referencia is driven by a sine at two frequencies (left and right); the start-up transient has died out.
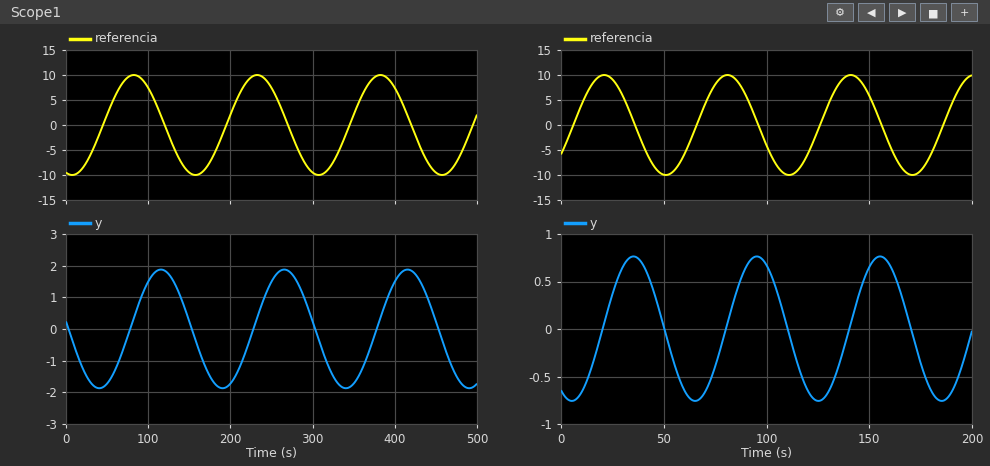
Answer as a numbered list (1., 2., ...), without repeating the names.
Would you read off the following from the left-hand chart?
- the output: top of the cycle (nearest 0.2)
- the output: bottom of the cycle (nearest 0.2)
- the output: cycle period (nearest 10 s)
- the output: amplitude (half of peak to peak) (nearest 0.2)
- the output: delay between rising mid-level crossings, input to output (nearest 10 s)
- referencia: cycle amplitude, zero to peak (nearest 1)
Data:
1. 1.8
2. -1.8
3. 150 s
4. 1.8
5. 30 s
6. 10
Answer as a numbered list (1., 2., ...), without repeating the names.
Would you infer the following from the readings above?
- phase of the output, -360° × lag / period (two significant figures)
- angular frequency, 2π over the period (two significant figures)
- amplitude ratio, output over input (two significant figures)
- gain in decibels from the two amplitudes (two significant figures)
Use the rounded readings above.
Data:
1. -72°
2. 0.042 rad/s
3. 0.18
4. -15 dB
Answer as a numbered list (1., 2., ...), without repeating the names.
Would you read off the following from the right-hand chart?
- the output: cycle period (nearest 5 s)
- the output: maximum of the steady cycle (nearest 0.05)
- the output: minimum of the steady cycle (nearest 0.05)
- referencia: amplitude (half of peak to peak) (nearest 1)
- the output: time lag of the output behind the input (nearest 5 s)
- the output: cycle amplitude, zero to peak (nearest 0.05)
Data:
1. 60 s
2. 0.75
3. -0.75
4. 10
5. 15 s
6. 0.75
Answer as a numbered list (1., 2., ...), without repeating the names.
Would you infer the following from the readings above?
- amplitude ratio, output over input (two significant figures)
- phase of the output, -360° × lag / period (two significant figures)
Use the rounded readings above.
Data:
1. 0.075
2. -90°
